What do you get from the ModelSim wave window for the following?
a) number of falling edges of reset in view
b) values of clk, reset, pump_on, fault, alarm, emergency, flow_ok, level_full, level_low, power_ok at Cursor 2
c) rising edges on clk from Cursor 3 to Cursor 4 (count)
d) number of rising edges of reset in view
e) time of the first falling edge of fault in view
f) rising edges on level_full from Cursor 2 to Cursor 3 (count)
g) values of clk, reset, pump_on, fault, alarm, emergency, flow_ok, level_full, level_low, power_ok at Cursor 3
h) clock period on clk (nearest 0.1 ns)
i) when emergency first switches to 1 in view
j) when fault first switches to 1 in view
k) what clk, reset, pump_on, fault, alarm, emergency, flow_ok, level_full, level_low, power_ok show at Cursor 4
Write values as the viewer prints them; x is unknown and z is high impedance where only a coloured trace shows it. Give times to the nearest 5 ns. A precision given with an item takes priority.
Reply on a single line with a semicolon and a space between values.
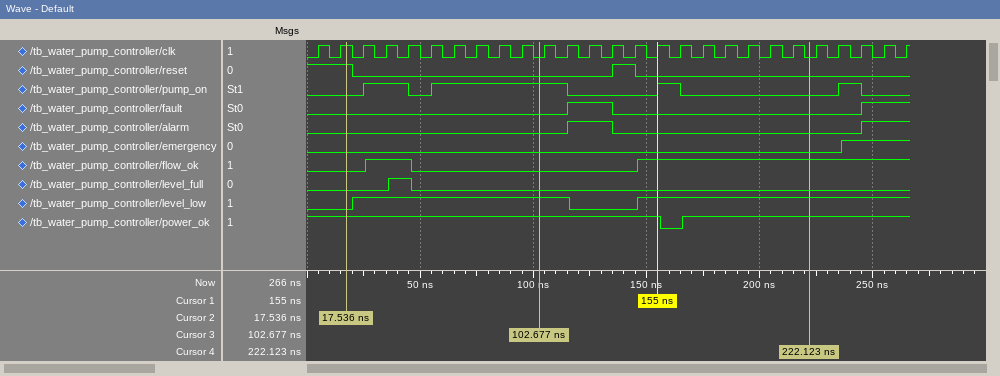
2; clk=1, reset=1, pump_on=0, fault=0, alarm=0, emergency=0, flow_ok=0, level_full=0, level_low=0, power_ok=1; 12; 1; 135 ns; 1; clk=0, reset=0, pump_on=1, fault=0, alarm=0, emergency=0, flow_ok=0, level_full=0, level_low=1, power_ok=1; 10 ns; 235 ns; 115 ns; clk=0, reset=0, pump_on=0, fault=0, alarm=0, emergency=0, flow_ok=1, level_full=0, level_low=1, power_ok=1
